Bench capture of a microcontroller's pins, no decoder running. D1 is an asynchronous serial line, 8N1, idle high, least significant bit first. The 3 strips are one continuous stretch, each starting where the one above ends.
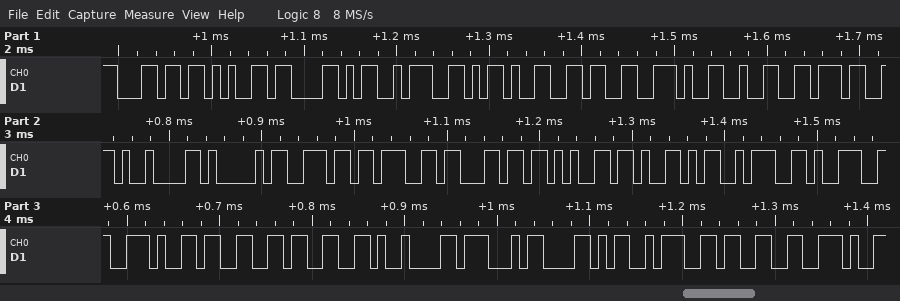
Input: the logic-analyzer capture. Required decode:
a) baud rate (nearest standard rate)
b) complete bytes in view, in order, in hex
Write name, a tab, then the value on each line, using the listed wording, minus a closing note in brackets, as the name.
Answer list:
baud rate	115200 baud
complete bytes in view, in order, in hex	6C 65 58 3A 2D 36 2E 32 37 09 41 6E 67 6C 65 59 3A 39 2E 33 33 09 47 58 3A 33 2E
